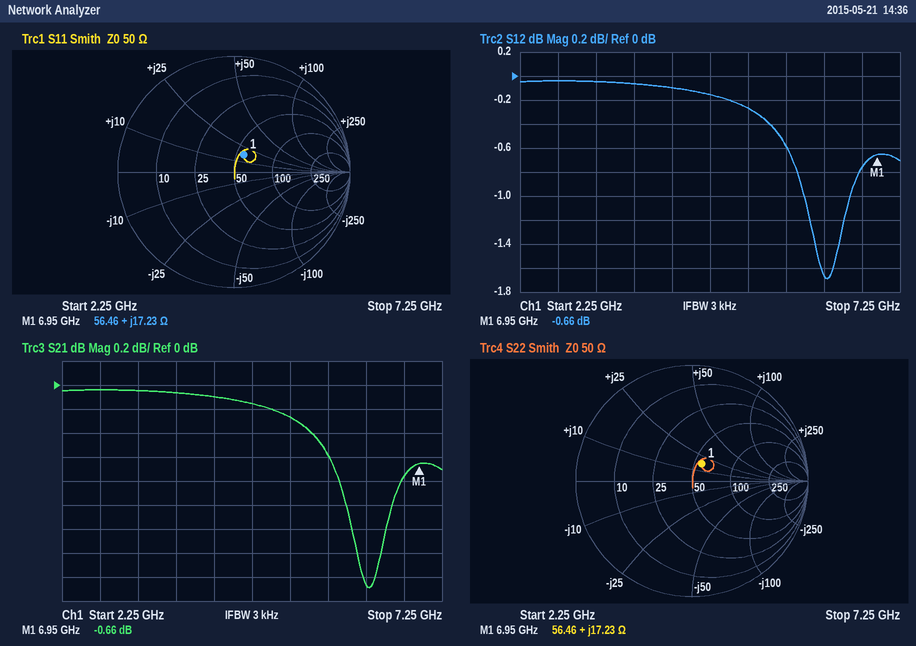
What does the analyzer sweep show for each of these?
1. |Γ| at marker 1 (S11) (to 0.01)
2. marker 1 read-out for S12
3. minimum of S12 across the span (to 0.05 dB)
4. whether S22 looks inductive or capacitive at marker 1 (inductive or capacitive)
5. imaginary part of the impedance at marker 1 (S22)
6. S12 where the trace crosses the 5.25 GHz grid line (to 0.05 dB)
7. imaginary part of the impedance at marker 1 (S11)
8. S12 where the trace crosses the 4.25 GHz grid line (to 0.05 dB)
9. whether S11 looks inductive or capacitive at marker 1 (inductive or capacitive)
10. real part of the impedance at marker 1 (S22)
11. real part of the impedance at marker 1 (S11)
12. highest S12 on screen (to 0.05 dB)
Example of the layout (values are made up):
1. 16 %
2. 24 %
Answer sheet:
1. 0.17
2. -0.66 dB
3. -1.70 dB
4. inductive
5. +17.23 Ω
6. -0.25 dB
7. +17.23 Ω
8. -0.10 dB
9. inductive
10. 56.46 Ω
11. 56.46 Ω
12. -0.05 dB
